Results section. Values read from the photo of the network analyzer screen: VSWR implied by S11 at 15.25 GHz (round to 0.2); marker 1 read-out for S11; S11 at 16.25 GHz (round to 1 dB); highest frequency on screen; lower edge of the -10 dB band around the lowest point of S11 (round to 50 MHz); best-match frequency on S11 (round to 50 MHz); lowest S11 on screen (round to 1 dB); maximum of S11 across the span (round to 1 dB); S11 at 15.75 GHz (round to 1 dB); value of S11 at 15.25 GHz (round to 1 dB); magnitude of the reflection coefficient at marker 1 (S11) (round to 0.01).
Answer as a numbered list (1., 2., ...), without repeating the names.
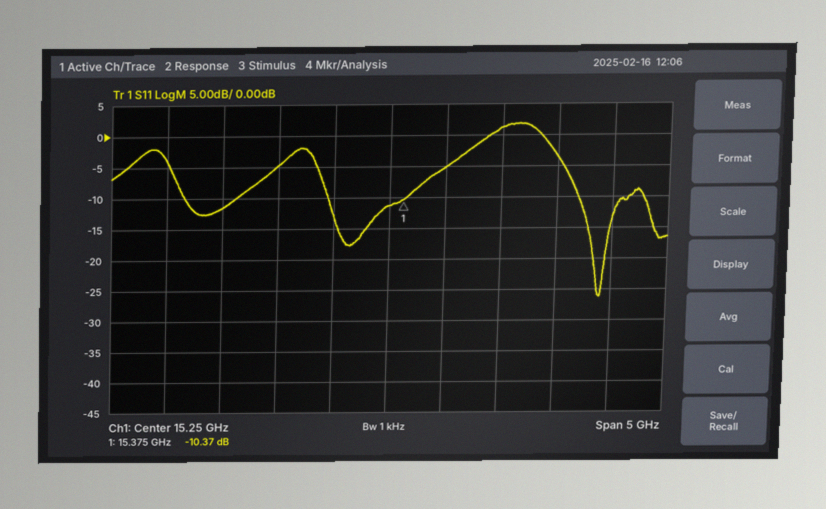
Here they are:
1. 1.8
2. -10.37 dB
3. 1 dB
4. 17.75 GHz
5. 16.95 GHz
6. 17.15 GHz
7. -26 dB
8. 2 dB
9. -5 dB
10. -11 dB
11. 0.30
